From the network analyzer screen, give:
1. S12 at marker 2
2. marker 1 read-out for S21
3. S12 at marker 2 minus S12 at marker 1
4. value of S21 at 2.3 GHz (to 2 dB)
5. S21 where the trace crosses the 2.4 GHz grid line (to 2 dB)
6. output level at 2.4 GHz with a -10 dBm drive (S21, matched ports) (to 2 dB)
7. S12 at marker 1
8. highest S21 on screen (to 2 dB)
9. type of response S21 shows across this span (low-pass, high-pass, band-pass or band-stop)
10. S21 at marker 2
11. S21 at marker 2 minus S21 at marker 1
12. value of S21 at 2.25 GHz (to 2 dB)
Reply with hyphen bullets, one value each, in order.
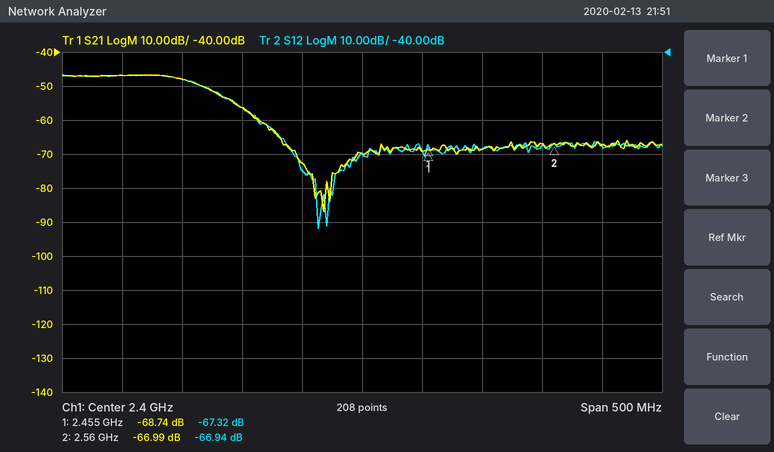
- -66.94 dB
- -68.74 dB
- 0.38 dB
- -56 dB
- -70 dB
- -80 dBm
- -67.32 dB
- -46 dB
- low-pass
- -66.99 dB
- 1.75 dB
- -48 dB
